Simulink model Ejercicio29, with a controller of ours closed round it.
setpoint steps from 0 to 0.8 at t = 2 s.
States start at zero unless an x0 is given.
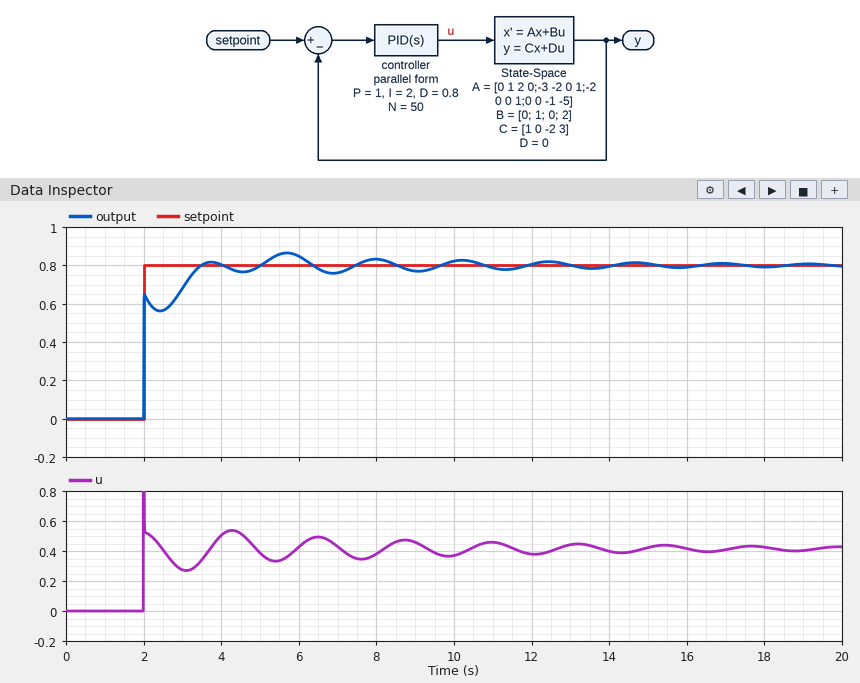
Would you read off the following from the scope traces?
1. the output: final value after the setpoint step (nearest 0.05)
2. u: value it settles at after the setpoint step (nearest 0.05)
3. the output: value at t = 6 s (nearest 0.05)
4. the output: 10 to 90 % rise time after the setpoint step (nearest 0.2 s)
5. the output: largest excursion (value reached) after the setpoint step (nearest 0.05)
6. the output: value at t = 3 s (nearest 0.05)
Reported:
0.80
0.40
0.85
1.2 s
0.85
0.70
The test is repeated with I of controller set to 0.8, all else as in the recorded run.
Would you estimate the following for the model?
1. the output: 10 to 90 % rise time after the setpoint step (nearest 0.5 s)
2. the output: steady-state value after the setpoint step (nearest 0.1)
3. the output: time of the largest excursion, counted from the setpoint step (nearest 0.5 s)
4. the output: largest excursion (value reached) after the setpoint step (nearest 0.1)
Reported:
3.0 s
0.8
6.0 s
0.8
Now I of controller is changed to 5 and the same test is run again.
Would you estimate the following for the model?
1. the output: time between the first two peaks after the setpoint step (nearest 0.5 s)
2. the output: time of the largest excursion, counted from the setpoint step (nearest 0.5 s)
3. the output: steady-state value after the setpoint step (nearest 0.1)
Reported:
2.5 s
1.5 s
0.8
